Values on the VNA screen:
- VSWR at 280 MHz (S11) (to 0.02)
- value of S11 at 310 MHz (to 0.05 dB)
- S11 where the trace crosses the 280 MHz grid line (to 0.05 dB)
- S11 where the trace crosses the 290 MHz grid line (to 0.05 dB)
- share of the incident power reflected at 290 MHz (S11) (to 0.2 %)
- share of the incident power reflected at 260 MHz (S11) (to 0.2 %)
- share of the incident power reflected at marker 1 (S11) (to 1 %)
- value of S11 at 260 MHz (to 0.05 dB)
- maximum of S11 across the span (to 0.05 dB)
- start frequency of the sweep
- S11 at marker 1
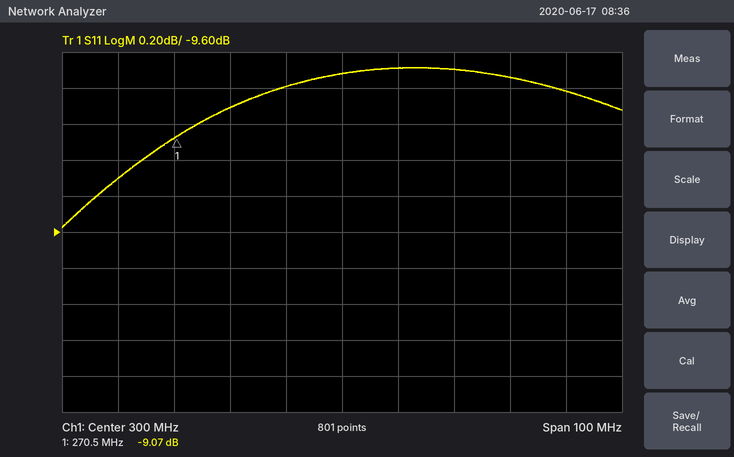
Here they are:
2.12
-8.70 dB
-8.90 dB
-8.80 dB
13.2 %
11.8 %
12 %
-9.30 dB
-8.70 dB
250 MHz
-9.07 dB
